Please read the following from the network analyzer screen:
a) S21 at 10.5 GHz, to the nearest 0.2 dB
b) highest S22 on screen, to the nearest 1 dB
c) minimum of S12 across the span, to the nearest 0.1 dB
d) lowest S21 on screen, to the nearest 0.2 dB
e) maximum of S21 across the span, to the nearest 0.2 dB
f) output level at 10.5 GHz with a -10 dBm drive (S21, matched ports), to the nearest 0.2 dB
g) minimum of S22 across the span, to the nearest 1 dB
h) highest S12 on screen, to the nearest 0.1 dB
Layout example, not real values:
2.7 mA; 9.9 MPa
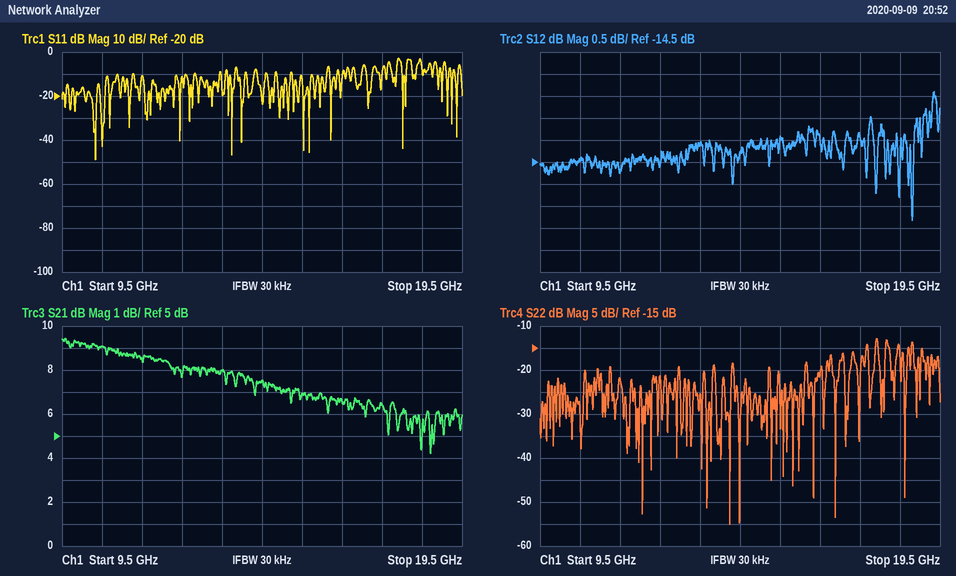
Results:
9.0 dB; -13 dB; -15.8 dB; 4.2 dB; 9.4 dB; -1.0 dBm; -55 dB; -12.9 dB
